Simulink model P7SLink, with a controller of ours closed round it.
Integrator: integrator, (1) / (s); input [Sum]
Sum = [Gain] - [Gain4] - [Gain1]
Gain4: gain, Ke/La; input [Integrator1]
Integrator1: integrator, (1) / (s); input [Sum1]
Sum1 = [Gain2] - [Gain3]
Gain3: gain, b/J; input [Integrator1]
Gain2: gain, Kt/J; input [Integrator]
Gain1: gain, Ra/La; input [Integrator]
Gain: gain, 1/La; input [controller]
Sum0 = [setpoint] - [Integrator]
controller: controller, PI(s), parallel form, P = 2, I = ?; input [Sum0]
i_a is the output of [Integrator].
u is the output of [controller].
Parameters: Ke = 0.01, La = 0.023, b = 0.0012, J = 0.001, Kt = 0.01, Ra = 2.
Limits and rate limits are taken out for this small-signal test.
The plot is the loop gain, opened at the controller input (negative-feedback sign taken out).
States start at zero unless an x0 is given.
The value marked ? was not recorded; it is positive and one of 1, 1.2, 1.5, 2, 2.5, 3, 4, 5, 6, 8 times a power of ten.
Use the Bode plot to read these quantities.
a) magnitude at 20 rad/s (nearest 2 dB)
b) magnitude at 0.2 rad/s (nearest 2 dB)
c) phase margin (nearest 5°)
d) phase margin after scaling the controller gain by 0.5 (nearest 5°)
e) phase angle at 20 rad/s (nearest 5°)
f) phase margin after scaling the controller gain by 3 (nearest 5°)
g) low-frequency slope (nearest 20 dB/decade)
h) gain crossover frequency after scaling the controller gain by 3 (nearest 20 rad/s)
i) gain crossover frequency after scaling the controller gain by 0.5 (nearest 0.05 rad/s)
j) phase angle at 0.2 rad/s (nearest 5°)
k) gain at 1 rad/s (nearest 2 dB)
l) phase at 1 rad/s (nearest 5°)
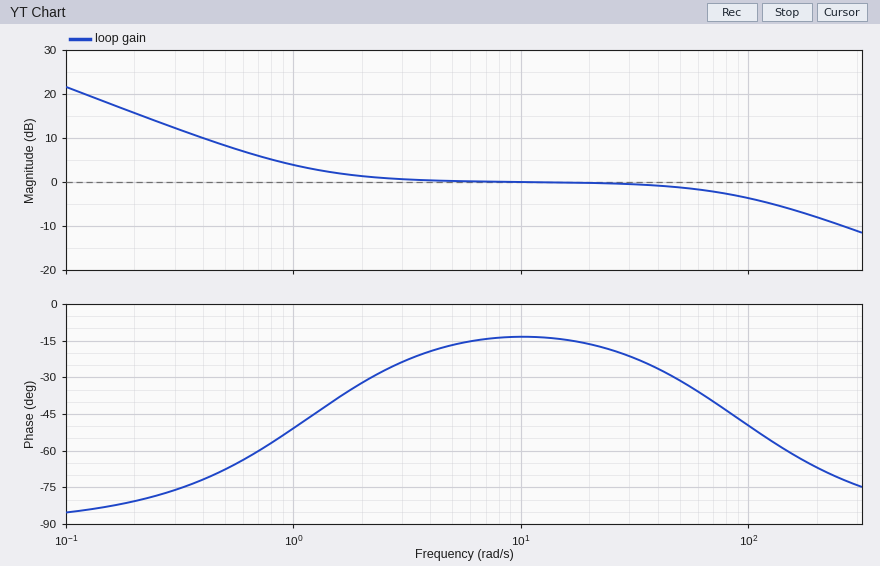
0 dB
16 dB
165°
120°
-15°
110°
-20 dB/decade
240 rad/s
0.70 rad/s
-80°
4 dB
-50°
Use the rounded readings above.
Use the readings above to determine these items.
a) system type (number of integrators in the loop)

1
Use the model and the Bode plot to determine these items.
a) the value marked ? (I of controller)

2.5
